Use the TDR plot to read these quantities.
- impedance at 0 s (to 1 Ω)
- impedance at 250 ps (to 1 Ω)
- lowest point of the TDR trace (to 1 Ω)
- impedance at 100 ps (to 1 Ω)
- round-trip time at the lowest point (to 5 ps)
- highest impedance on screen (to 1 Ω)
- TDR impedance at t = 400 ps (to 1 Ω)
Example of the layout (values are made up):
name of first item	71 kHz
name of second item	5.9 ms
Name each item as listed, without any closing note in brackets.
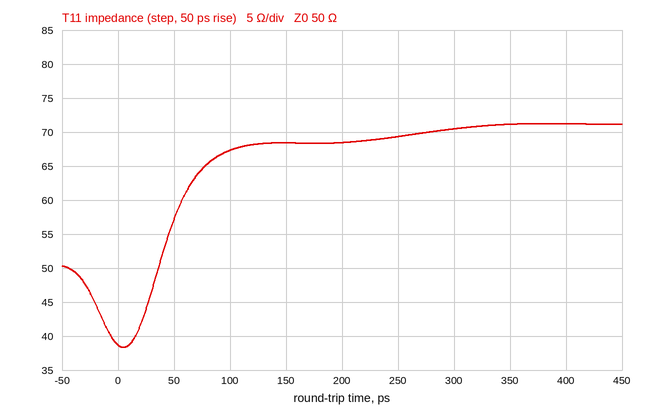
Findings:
impedance at 0 s	39 Ω
impedance at 250 ps	69 Ω
lowest point of the TDR trace	38 Ω
impedance at 100 ps	67 Ω
round-trip time at the lowest point	5 ps
highest impedance on screen	71 Ω
TDR impedance at t = 400 ps	71 Ω
